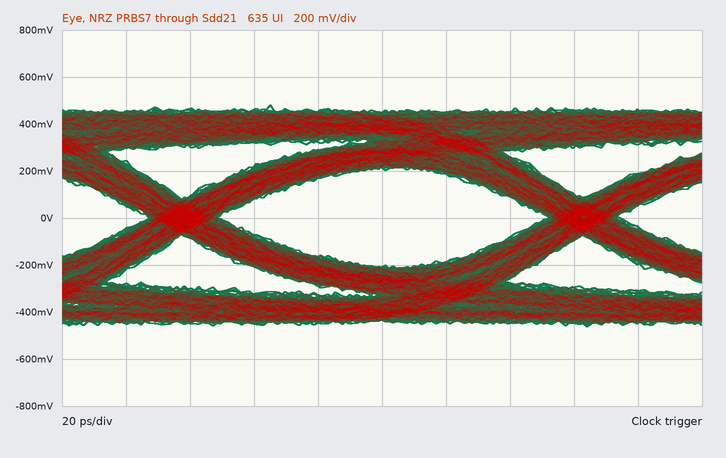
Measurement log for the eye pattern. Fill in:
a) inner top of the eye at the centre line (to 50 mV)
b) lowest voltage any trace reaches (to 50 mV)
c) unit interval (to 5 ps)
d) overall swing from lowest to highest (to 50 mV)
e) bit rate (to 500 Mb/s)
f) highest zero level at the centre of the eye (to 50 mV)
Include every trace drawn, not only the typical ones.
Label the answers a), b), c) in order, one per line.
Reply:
a) 200 mV
b) -450 mV
c) 125 ps
d) 950 mV
e) 8.0 Gb/s
f) -200 mV
